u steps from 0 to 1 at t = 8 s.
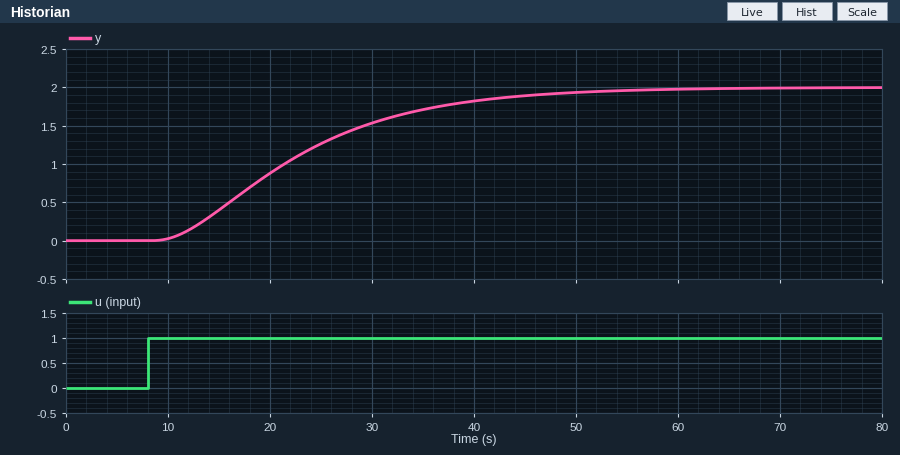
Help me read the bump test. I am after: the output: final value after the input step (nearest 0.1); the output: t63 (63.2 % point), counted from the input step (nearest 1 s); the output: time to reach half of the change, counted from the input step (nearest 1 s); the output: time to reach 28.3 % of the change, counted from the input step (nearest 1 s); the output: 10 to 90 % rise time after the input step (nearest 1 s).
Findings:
2.0
17 s
13 s
9 s
26 s
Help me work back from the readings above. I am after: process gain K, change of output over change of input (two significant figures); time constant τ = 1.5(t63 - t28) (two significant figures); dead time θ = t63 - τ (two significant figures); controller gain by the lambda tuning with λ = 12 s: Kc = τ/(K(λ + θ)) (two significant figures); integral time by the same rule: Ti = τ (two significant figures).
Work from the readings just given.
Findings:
2.0
12 s
5.0 s
0.35
12 s
